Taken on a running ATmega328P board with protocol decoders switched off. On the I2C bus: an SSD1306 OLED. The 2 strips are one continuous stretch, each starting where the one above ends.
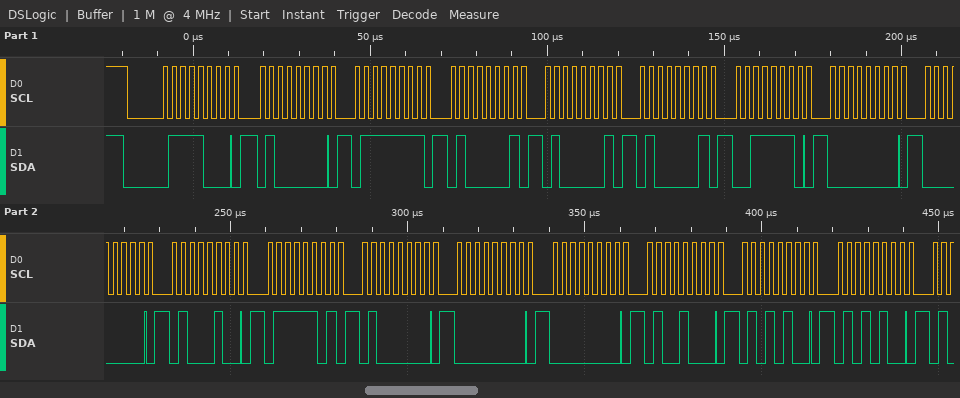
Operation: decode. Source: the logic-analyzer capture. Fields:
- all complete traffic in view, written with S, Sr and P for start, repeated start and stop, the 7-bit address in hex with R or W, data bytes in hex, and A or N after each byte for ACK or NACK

S 3CW A 40 A 7F A 41 A 41 A 41 A 3E A 00 A 00 A 44 A 7D A 40 A 00 A 00 A 48 A 54 A 54 A
